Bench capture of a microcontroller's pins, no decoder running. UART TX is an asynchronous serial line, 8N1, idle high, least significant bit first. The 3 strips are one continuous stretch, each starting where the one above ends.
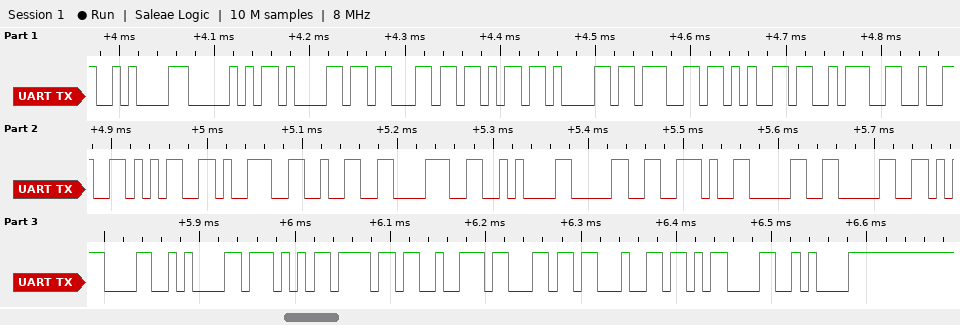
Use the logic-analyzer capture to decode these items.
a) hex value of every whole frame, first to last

0A 50 61 63 6B 61 67 65 3A 32 35 39 32 38 0A 30 2E 30 30 0D 0A 57 6F 72 6C 64 0D 0A
